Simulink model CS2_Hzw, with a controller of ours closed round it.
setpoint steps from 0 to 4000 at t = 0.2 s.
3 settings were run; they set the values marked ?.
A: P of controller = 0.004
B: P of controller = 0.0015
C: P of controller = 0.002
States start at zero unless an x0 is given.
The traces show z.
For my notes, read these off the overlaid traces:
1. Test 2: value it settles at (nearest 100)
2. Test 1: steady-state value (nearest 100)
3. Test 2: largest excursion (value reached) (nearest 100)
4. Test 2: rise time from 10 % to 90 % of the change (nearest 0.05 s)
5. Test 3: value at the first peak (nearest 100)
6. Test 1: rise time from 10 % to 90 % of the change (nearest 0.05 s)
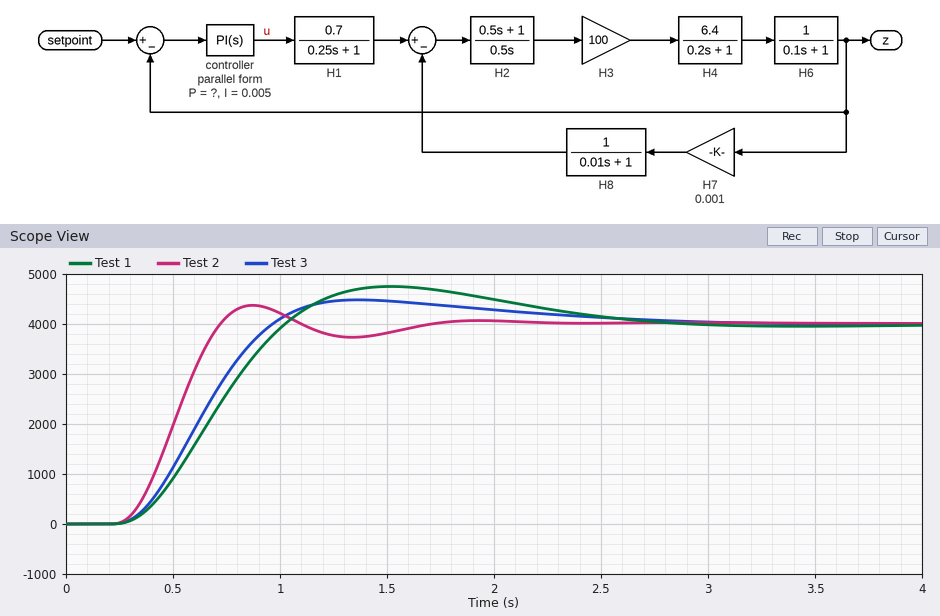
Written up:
4000
4000
4400
0.30 s
4500
0.50 s
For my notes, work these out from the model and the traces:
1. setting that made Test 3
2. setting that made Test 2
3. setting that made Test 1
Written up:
C
A
B
